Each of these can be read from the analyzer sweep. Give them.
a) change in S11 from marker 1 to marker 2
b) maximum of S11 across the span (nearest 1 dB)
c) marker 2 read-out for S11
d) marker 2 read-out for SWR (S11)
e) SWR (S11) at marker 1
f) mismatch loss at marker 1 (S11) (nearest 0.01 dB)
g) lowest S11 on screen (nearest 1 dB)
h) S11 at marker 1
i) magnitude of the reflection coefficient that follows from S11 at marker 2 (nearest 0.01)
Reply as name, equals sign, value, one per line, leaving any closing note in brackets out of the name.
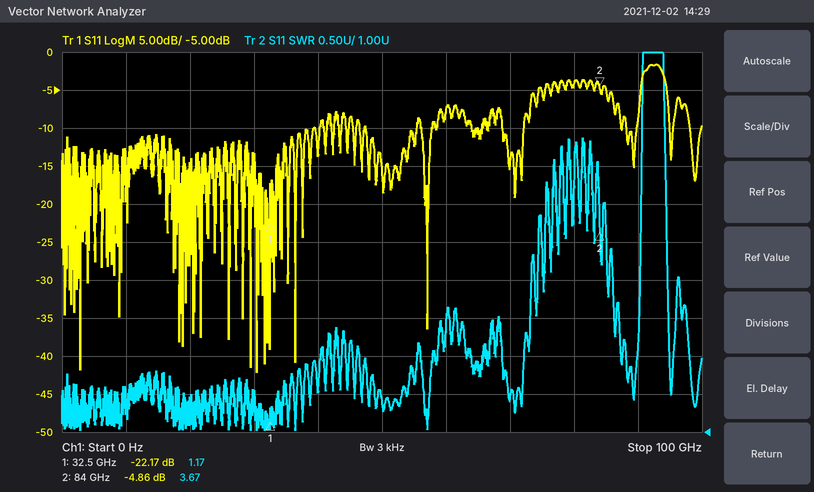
change in S11 from marker 1 to marker 2 = 17.31 dB
maximum of S11 across the span = -2 dB
marker 2 read-out for S11 = -4.86 dB
marker 2 read-out for SWR = 3.67
SWR (S11) at marker 1 = 1.17
mismatch loss at marker 1 (S11) = 0.03 dB
lowest S11 on screen = -42 dB
S11 at marker 1 = -22.17 dB
magnitude of the reflection coefficient that follows from S11 at marker 2 = 0.57
